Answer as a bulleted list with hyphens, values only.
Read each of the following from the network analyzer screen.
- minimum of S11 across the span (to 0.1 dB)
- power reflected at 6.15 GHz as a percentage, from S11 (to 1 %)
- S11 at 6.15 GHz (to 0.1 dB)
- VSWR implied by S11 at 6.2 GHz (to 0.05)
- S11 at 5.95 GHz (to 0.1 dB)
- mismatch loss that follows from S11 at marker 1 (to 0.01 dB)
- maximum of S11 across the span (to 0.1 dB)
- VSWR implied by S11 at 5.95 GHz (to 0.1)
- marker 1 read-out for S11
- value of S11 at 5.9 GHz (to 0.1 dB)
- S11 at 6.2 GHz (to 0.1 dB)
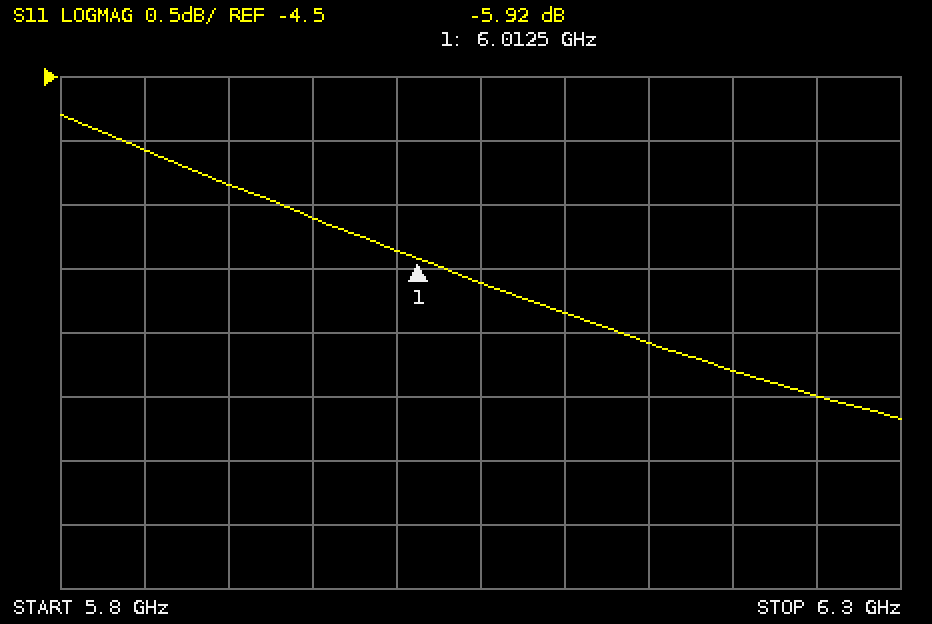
- -7.2 dB
- 22 %
- -6.6 dB
- 2.70
- -5.6 dB
- 1.28 dB
- -4.8 dB
- 3.2
- -5.92 dB
- -5.3 dB
- -6.8 dB
